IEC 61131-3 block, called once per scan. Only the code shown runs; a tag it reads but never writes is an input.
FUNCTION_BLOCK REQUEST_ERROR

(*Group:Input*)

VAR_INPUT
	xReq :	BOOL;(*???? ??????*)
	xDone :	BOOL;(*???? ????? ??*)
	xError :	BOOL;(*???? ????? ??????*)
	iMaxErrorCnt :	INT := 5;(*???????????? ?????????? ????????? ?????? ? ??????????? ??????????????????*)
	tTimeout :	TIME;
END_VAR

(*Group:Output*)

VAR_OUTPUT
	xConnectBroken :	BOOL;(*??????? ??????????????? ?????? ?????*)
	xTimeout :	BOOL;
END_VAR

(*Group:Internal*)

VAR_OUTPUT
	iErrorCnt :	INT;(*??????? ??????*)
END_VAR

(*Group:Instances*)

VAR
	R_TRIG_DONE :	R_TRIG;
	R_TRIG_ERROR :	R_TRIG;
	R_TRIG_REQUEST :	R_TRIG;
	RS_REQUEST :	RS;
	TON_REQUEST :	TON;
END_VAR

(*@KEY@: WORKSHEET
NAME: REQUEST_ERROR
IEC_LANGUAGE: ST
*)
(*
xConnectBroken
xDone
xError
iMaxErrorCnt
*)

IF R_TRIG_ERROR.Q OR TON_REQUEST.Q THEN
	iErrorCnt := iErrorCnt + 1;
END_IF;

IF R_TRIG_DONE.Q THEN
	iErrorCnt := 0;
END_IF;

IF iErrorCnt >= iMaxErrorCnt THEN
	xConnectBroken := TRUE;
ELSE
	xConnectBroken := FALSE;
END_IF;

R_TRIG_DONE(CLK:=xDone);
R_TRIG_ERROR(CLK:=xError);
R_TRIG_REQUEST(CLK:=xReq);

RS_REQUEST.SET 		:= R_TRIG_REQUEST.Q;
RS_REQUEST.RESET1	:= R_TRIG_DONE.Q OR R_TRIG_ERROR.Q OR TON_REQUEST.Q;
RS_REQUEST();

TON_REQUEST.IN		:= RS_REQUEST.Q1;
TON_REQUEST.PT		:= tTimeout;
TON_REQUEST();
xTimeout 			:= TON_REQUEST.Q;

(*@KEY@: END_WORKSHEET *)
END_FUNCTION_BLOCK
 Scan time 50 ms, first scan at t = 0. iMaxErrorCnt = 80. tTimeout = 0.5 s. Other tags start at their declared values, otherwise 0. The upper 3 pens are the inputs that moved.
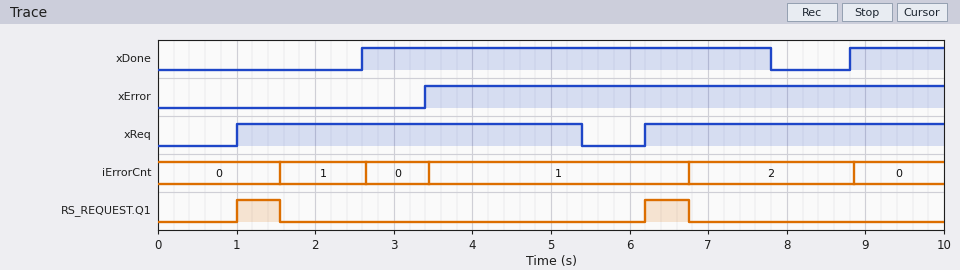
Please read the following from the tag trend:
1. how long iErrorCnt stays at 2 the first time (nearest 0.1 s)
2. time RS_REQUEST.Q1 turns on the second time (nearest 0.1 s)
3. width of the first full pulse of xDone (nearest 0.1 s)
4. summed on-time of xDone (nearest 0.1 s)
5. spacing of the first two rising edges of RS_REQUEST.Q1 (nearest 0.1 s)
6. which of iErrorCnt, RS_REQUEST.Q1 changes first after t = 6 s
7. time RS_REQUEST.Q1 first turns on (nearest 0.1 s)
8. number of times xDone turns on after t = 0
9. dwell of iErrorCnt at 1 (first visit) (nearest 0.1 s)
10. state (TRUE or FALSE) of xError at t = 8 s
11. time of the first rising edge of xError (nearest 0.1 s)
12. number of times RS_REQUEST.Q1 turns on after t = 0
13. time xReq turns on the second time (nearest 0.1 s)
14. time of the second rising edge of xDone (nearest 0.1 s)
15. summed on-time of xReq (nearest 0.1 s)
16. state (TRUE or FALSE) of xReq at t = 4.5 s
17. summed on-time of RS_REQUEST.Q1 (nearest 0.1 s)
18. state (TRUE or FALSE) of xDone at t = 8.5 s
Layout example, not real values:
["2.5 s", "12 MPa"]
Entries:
["2.1 s", "6.2 s", "5.2 s", "6.4 s", "5.2 s", "RS_REQUEST.Q1", "1.0 s", "2", "1.1 s", "TRUE", "3.4 s", "2", "6.2 s", "8.8 s", "8.2 s", "TRUE", "1.1 s", "FALSE"]
